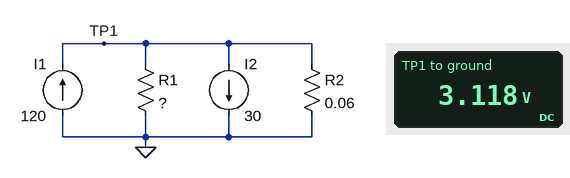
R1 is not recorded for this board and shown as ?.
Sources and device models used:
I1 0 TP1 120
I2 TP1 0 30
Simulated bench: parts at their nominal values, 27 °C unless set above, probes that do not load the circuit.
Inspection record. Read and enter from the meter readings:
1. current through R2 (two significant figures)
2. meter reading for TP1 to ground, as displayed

52 A
3.118 V
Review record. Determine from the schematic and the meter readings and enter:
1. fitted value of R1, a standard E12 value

0.082 Ω
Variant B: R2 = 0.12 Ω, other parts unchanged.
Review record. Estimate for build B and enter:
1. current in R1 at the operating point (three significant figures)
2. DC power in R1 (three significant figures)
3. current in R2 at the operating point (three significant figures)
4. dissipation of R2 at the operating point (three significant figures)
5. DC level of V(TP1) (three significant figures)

53.5 A
234 W
36.5 A
160 W
4.38 V
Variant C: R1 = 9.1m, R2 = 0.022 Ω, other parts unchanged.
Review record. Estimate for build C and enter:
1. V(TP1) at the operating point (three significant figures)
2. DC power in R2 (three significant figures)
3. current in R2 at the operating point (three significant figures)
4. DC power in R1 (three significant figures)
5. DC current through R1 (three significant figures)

579 mV
15.3 W
26.3 A
36.9 W
63.7 A
